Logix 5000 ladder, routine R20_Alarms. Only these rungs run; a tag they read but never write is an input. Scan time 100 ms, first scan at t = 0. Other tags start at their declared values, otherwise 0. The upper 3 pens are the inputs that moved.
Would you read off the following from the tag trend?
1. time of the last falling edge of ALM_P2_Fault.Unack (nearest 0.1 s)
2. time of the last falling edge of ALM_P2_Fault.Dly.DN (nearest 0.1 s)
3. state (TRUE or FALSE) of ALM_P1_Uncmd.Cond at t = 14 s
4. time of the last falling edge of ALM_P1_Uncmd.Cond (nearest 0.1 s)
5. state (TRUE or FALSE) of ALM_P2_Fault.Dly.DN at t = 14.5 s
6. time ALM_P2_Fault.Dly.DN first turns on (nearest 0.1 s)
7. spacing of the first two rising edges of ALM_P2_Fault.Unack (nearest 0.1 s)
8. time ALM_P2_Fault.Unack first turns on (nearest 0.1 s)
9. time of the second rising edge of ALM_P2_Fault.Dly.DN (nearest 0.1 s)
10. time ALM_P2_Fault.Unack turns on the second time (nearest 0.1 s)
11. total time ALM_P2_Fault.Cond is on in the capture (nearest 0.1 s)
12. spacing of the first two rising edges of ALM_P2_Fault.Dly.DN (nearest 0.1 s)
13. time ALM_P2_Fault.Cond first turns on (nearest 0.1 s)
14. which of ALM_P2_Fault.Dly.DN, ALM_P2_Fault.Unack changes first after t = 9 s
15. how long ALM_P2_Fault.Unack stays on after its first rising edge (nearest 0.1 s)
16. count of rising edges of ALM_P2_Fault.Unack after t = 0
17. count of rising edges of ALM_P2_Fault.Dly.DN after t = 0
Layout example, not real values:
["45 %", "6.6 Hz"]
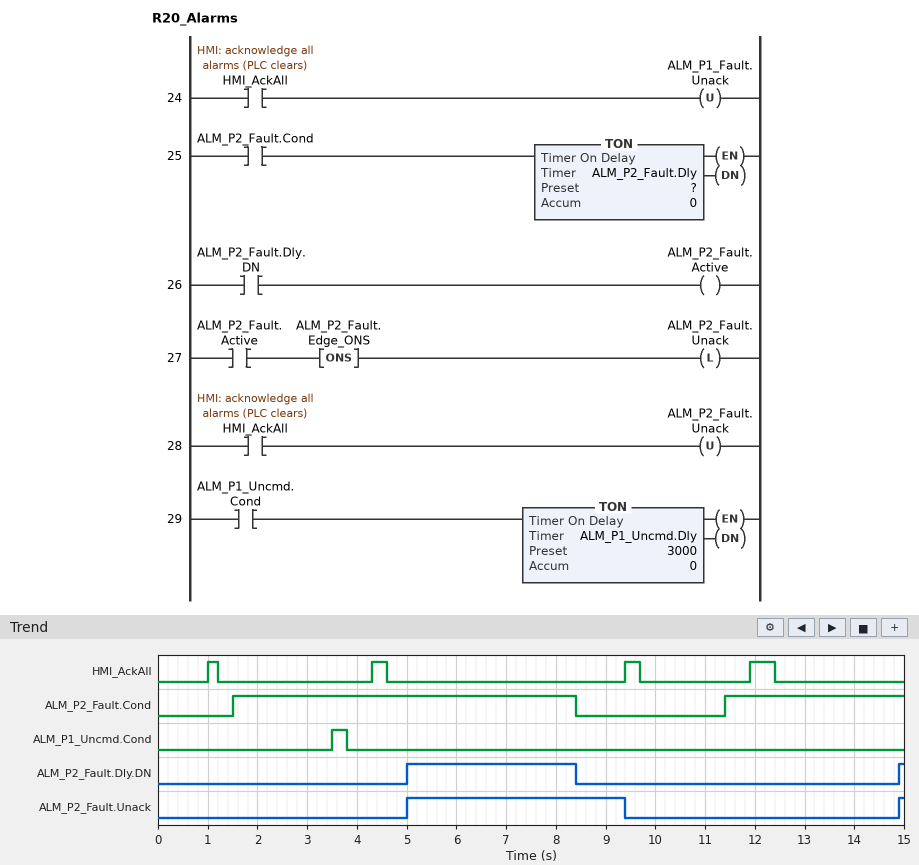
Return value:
["9.4 s", "8.4 s", "FALSE", "3.8 s", "FALSE", "5.0 s", "9.9 s", "5.0 s", "14.9 s", "14.9 s", "10.5 s", "9.9 s", "1.5 s", "ALM_P2_Fault.Unack", "4.4 s", "2", "2"]
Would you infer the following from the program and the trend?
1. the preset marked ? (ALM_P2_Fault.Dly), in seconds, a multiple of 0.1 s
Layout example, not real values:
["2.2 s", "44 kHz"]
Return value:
["3.5 s"]
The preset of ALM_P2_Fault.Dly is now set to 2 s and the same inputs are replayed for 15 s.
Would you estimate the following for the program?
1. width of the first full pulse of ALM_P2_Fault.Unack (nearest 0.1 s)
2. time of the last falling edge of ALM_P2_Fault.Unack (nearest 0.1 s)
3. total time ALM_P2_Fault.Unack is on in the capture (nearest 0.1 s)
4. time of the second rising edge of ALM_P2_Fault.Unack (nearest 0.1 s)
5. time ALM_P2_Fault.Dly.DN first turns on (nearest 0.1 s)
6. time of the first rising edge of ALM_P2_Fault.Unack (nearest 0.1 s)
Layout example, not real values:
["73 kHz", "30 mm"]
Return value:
["0.8 s", "4.3 s", "2.4 s", "13.4 s", "3.5 s", "3.5 s"]
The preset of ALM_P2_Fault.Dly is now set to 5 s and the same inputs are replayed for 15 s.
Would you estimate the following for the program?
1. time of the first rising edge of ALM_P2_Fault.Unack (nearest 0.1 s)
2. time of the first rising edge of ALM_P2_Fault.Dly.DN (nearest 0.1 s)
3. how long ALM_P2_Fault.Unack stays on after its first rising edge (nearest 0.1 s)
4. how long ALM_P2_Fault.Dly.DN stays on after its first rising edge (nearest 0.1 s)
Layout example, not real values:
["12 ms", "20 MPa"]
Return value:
["6.5 s", "6.5 s", "2.9 s", "1.9 s"]
